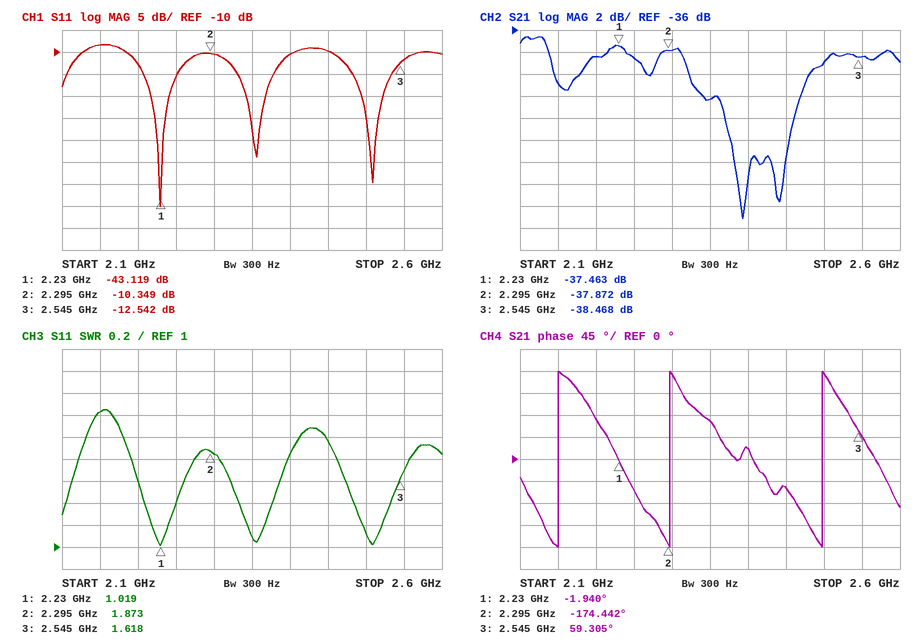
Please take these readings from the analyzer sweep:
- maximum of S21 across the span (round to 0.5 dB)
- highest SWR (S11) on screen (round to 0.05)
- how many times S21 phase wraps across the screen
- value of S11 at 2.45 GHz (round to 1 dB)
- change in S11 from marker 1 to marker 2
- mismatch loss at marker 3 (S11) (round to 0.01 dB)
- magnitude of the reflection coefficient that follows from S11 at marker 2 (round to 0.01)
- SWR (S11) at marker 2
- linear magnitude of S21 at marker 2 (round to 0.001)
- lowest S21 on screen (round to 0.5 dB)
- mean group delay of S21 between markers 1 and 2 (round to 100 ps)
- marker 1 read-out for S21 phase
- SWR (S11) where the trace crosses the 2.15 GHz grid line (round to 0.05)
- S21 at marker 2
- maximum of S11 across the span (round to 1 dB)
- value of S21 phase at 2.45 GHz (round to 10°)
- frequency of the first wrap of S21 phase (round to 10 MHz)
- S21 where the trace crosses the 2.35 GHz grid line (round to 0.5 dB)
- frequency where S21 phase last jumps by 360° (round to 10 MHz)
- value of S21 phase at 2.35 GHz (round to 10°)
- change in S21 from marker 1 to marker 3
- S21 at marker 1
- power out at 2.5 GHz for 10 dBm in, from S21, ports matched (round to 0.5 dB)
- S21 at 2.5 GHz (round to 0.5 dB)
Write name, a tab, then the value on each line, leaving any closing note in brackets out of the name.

maximum of S21 across the span	-36.5 dB
highest SWR (S11) on screen	2.25
how many times S21 phase wraps across the screen	3
value of S11 at 2.45 GHz	-10 dB
change in S11 from marker 1 to marker 2	32.770 dB
mismatch loss at marker 3 (S11)	0.25 dB
magnitude of the reflection coefficient that follows from S11 at marker 2	0.30
SWR (S11) at marker 2	1.873
linear magnitude of S21 at marker 2	0.013
lowest S21 on screen	-53.0 dB
mean group delay of S21 between markers 1 and 2	7.4 ns
marker 1 read-out for S21 phase	-1.940°
SWR (S11) where the trace crosses the 2.15 GHz grid line	2.25
S21 at marker 2	-37.872 dB
maximum of S11 across the span	-8 dB
value of S21 phase at 2.45 GHz	-60°
frequency of the first wrap of S21 phase	2.15 GHz
S21 where the trace crosses the 2.35 GHz grid line	-42.5 dB
frequency where S21 phase last jumps by 360°	2.50 GHz
value of S21 phase at 2.35 GHz	80°
change in S21 from marker 1 to marker 3	-1.005 dB
S21 at marker 1	-37.463 dB
power out at 2.5 GHz for 10 dBm in, from S21, ports matched	-29.0 dBm
S21 at 2.5 GHz	-39.0 dB
